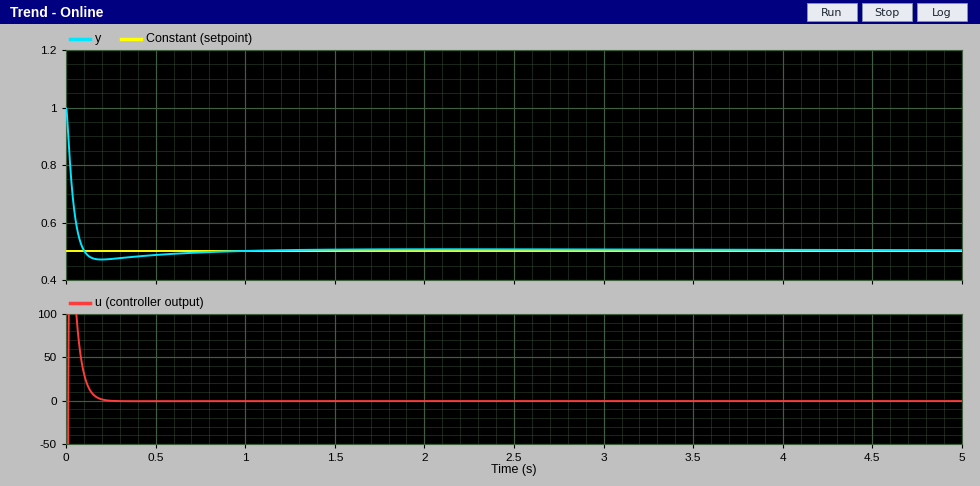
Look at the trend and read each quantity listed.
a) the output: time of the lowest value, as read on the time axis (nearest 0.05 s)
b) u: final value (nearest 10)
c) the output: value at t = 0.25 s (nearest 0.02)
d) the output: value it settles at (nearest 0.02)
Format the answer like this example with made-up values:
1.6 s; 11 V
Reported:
0.20 s; 0; 0.48; 0.50
